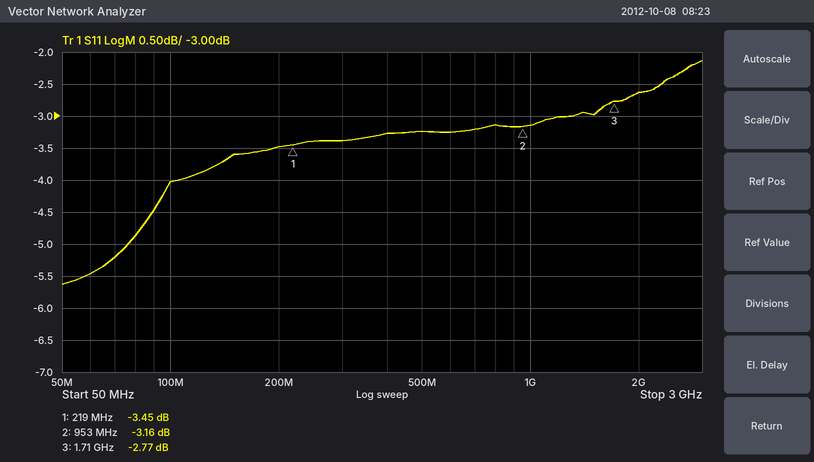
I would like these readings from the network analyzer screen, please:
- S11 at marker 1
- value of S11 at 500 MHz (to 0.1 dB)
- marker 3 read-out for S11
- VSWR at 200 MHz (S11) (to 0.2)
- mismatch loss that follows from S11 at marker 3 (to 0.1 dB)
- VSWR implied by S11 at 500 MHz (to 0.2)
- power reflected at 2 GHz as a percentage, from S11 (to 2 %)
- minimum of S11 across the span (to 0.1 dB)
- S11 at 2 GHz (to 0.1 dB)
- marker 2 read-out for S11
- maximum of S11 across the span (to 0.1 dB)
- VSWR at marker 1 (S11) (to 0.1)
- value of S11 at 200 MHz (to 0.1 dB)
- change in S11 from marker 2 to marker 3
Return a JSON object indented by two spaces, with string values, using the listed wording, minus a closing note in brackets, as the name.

{
  "S11 at marker 1": "-3.45 dB",
  "value of S11 at 500 MHz": "-3.2 dB",
  "marker 3 read-out for S11": "-2.77 dB",
  "VSWR at 200 MHz (S11)": "5.0",
  "mismatch loss that follows from S11 at marker 3": "3.3 dB",
  "VSWR implied by S11 at 500 MHz": "5.4",
  "power reflected at 2 GHz as a percentage, from S11": "54 %",
  "minimum of S11 across the span": "-5.6 dB",
  "S11 at 2 GHz": "-2.6 dB",
  "marker 2 read-out for S11": "-3.16 dB",
  "maximum of S11 across the span": "-2.1 dB",
  "VSWR at marker 1 (S11)": "5.1",
  "value of S11 at 200 MHz": "-3.5 dB",
  "change in S11 from marker 2 to marker 3": "0.39 dB"
}
